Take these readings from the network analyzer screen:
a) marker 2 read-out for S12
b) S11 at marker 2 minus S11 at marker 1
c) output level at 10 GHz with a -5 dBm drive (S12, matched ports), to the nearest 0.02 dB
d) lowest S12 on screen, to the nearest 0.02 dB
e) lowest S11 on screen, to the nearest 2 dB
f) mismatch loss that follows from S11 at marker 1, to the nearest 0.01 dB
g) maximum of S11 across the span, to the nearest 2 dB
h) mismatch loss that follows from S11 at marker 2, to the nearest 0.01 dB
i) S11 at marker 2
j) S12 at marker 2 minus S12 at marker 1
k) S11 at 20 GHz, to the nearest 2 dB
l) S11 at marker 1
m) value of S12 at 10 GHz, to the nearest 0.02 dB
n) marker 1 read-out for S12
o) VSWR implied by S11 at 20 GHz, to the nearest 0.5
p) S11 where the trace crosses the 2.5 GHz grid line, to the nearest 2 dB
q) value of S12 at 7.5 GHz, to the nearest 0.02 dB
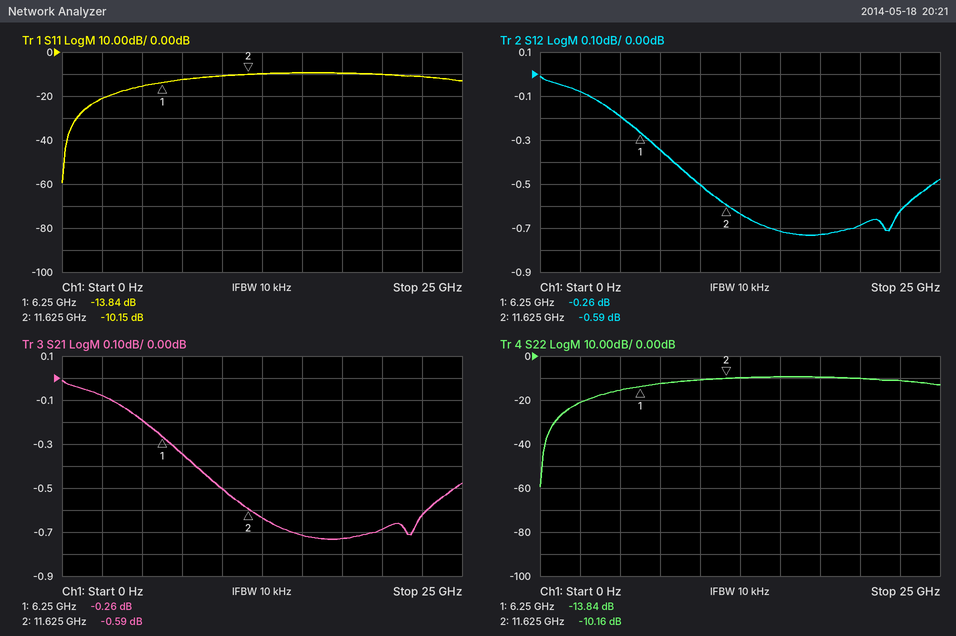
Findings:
-0.59 dB
3.69 dB
-5.50 dBm
-0.74 dB
-60 dB
0.18 dB
-10 dB
0.44 dB
-10.15 dB
-0.33 dB
-10 dB
-13.84 dB
-0.50 dB
-0.26 dB
2.0
-22 dB
-0.34 dB
